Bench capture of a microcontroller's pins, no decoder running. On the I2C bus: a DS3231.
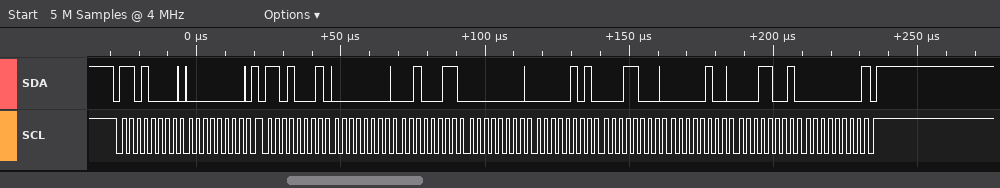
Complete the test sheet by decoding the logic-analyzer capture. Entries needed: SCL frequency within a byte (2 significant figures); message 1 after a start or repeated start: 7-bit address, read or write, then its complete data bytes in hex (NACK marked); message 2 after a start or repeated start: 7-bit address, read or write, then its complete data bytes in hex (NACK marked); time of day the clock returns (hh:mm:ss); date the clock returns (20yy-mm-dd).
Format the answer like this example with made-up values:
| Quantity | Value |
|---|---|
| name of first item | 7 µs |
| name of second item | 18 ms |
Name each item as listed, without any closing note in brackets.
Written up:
| Quantity | Value |
|---|---|
| SCL frequency within a byte | 400 kHz |
| message 1 after a start or repeated start: 7-bit address, read or write, then its complete data bytes in hex | 0x68 write: 00 |
| message 2 after a start or repeated start: 7-bit address, read or write, then its complete data bytes in hex | 0x68 read: 00 23 00 05 18 04 19 00 NACK |
| time of day the clock returns | 00:23:00 |
| date the clock returns | 2019-04-18 |
